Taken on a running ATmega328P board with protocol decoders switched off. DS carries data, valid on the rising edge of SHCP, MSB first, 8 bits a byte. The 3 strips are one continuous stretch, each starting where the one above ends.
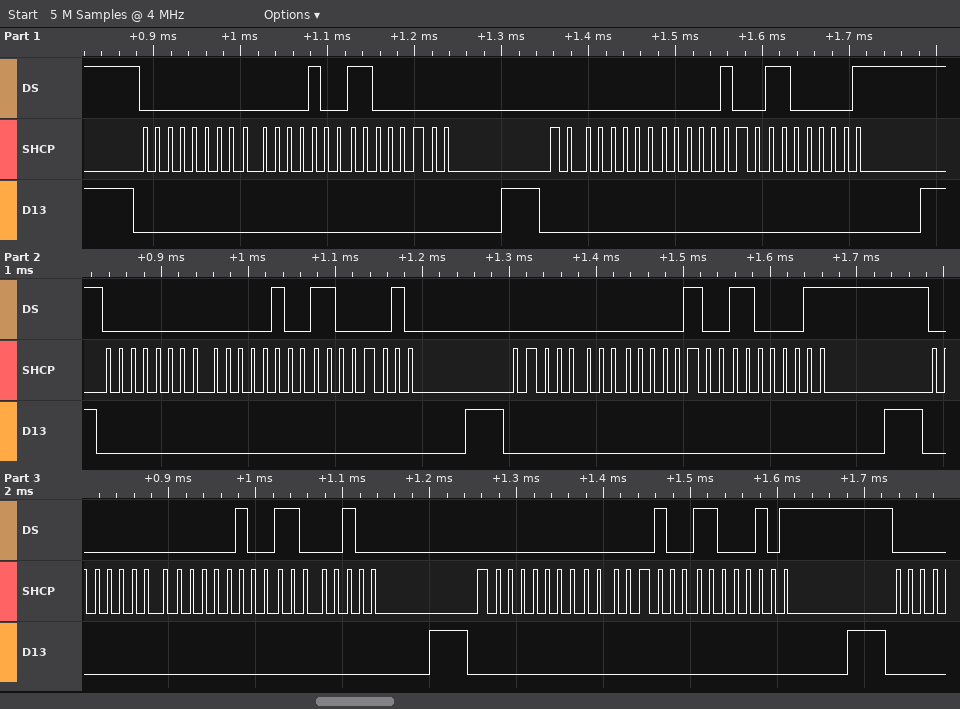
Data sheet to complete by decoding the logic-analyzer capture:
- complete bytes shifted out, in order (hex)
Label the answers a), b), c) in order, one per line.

a) 00 04 C0 00 04 C1 00 04 C2 00 04 C3 00 04 C4 00 04 C5
